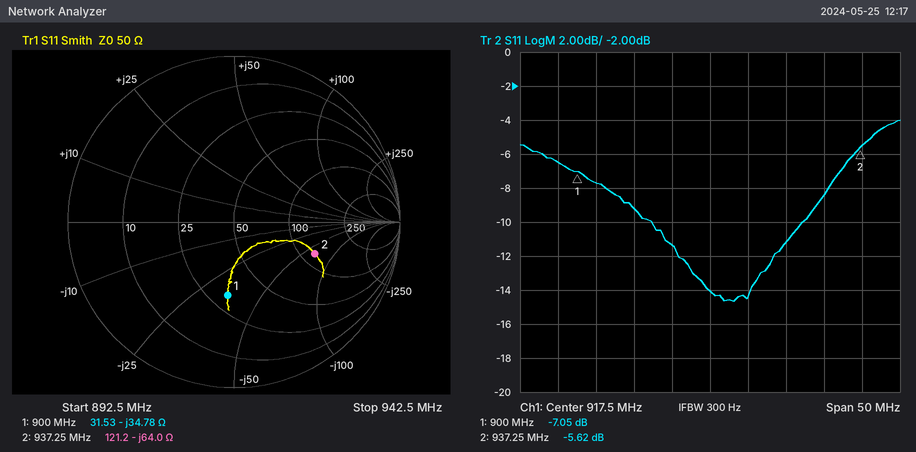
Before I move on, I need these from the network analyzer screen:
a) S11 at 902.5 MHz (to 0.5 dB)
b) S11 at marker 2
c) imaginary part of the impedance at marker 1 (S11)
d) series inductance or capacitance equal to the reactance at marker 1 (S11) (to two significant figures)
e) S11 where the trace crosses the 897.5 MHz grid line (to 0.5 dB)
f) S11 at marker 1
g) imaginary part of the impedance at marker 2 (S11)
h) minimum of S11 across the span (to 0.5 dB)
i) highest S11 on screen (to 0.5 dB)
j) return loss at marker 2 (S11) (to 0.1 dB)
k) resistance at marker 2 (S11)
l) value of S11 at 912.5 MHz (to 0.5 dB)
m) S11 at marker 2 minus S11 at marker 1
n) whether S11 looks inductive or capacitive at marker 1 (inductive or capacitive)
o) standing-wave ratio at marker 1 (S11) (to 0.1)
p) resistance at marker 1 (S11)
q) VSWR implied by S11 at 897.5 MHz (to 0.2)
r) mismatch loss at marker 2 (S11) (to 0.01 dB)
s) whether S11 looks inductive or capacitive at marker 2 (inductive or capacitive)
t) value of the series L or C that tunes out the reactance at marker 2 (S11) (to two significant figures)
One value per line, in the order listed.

-7.5 dB
-5.62 dB
-34.78 Ω
5.1 pF
-6.5 dB
-7.05 dB
-64.0 Ω
-14.5 dB
-4.0 dB
5.6 dB
121.2 Ω
-11.5 dB
1.43 dB
capacitive
2.6
31.53 Ω
2.8
1.39 dB
capacitive
11 nH
